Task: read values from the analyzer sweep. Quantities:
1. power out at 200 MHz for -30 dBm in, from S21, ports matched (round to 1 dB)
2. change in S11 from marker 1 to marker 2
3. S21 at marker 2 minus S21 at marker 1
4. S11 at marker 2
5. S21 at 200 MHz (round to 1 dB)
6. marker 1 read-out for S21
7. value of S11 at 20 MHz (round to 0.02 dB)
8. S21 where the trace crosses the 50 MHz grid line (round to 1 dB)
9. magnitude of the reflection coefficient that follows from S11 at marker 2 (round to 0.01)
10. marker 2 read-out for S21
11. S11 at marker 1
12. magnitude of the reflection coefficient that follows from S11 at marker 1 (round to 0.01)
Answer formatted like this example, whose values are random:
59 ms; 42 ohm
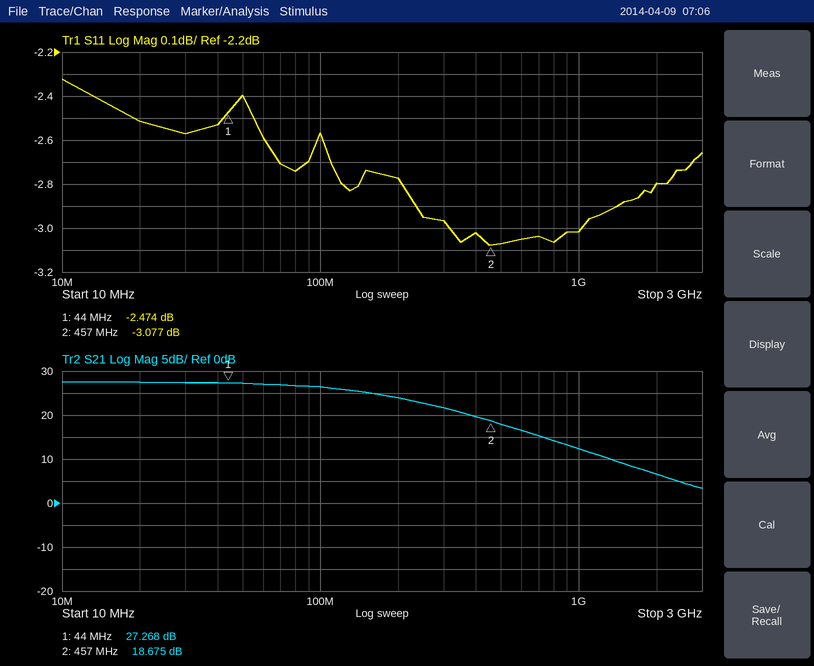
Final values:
-6 dBm; -0.603 dB; -8.593 dB; -3.077 dB; 24 dB; 27.268 dB; -2.52 dB; 27 dB; 0.70; 18.675 dB; -2.474 dB; 0.75
